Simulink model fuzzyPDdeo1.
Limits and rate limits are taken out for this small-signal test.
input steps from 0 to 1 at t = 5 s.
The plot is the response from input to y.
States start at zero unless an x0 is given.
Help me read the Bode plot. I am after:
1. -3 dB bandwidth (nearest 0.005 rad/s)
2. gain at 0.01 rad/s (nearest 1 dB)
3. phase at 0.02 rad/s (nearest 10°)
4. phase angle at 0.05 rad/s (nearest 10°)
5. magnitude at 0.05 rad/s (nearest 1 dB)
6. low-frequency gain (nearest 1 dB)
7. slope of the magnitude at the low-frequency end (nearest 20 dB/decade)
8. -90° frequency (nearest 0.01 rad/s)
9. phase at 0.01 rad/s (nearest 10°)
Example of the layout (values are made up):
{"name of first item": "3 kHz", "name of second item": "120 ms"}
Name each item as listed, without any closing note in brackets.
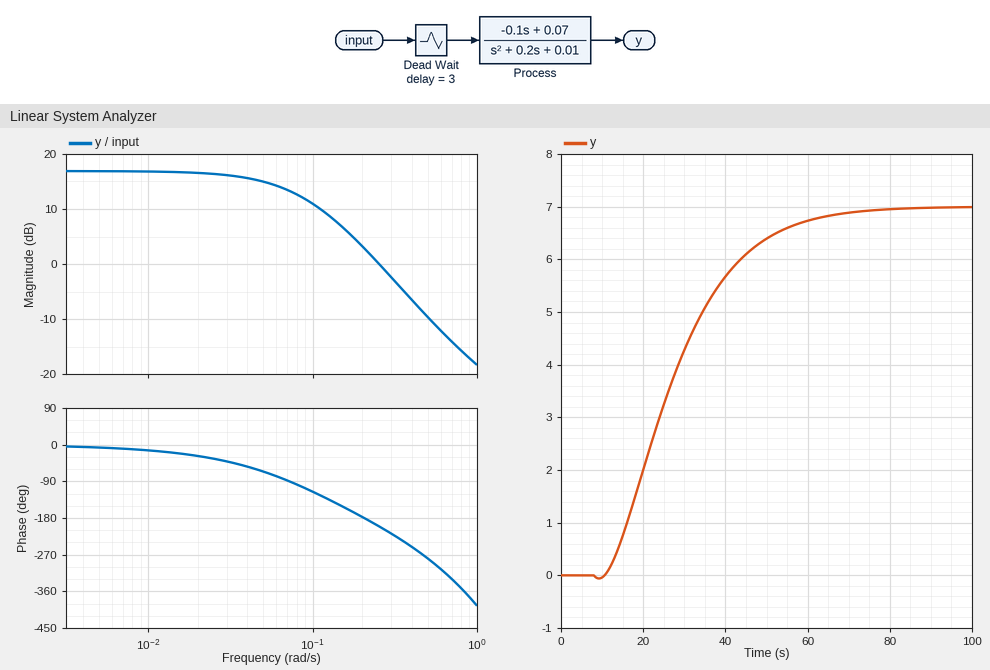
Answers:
{"-3 dB bandwidth": "0.065 rad/s", "gain at 0.01 rad/s": "17 dB", "phase at 0.02 rad/s": "-30°", "phase angle at 0.05 rad/s": "-70°", "magnitude at 0.05 rad/s": "15 dB", "low-frequency gain": "17 dB", "slope of the magnitude at the low-frequency end": "0 dB/decade", "-90° frequency": "0.07 rad/s", "phase at 0.01 rad/s": "-10°"}
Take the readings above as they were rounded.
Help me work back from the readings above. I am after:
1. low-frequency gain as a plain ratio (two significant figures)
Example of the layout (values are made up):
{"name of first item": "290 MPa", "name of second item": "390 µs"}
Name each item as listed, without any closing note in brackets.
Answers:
{"low-frequency gain as a plain ratio": "7.1"}
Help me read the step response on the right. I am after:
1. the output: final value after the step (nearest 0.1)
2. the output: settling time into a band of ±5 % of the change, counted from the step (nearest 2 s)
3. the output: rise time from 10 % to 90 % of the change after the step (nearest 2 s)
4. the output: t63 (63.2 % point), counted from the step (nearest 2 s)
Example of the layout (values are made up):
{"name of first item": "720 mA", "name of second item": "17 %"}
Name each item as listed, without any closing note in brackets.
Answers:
{"the output: final value after the step": "7.0", "the output: settling time into a band of ±5 % of the change, counted from the step": "52 s", "the output: rise time from 10 % to 90 % of the change after the step": "34 s", "the output: t63 (63.2 % point), counted from the step": "26 s"}
